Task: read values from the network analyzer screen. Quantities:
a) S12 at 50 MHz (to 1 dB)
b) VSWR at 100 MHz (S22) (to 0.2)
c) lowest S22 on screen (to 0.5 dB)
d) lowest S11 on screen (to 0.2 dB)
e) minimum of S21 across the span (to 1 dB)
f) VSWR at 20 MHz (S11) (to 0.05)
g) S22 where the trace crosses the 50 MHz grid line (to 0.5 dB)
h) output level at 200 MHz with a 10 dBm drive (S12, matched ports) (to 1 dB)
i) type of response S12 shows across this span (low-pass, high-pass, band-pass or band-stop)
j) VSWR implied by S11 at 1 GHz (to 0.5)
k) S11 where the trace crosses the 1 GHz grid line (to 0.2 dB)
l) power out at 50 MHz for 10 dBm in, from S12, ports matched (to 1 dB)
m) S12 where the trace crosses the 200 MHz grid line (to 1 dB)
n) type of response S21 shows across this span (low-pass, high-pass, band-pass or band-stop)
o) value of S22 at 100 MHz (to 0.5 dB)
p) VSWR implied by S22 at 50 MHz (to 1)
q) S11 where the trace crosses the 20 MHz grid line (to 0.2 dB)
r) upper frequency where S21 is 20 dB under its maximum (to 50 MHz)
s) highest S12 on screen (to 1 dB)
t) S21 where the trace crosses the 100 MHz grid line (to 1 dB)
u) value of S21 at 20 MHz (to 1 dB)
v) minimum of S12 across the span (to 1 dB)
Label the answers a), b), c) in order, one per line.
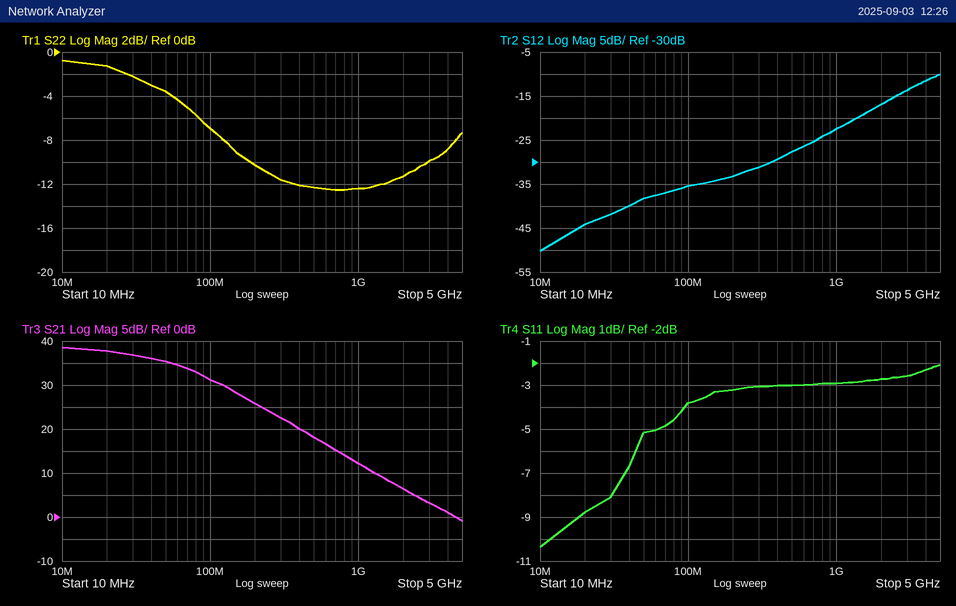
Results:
a) -38 dB
b) 2.6
c) -12.5 dB
d) -10.4 dB
e) -1 dB
f) 2.15
g) -3.5 dB
h) -23 dBm
i) high-pass
j) 6.0
k) -3.0 dB
l) -28 dBm
m) -33 dB
n) low-pass
o) -7.0 dB
p) 5
q) -8.8 dB
r) 500 MHz
s) -10 dB
t) 31 dB
u) 38 dB
v) -50 dB
